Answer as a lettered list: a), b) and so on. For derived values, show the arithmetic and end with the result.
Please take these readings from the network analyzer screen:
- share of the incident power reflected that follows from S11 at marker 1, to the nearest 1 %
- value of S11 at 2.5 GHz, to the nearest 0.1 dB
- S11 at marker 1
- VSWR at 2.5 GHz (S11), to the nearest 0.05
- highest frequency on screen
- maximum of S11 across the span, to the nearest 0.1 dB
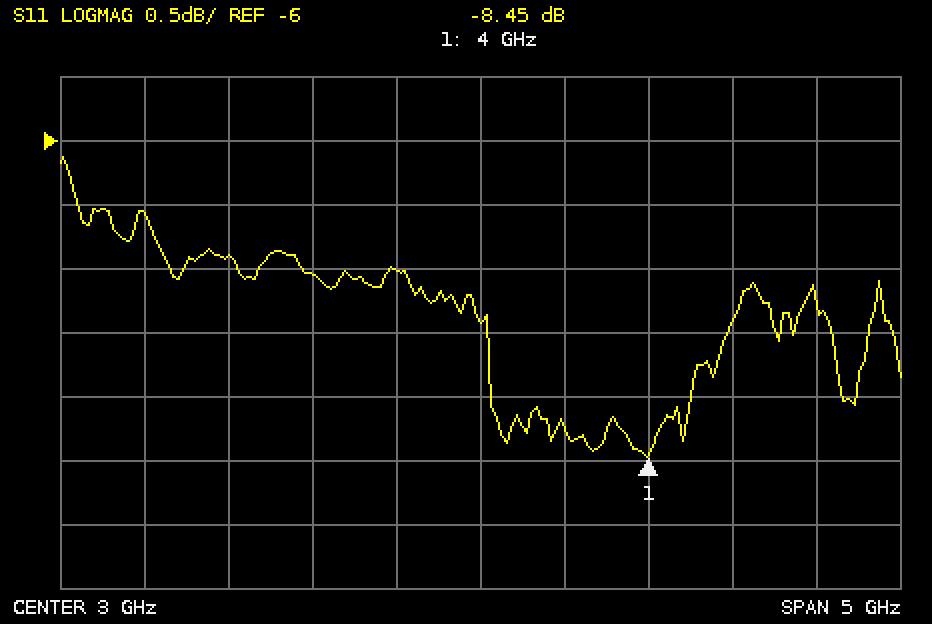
a) 10^(-8.45/10) ≈ 14 %
b) -7.0 dB
c) -8.45 dB
d) |Γ| = 10^(-7/20) = 0.4467; VSWR = (1 + 0.4467)/(1 − 0.4467) ≈ 2.61, so 2.60 to the nearest 0.05
e) 5.5 GHz
f) -6.1 dB
